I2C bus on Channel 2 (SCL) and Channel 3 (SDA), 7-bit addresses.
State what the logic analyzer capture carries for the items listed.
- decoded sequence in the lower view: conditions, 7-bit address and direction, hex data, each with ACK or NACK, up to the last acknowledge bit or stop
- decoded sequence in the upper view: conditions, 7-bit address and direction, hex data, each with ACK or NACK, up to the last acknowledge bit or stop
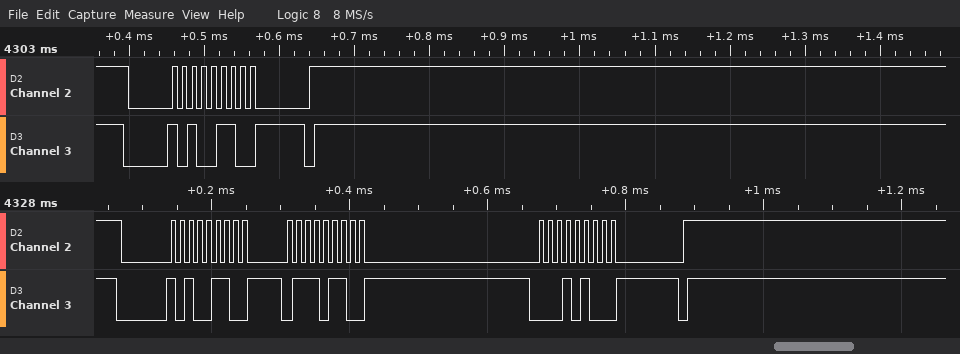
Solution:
start, address 53 write ACK, 76 ACK, 14 ACK, stop
start, address 53 write ACK, stop
